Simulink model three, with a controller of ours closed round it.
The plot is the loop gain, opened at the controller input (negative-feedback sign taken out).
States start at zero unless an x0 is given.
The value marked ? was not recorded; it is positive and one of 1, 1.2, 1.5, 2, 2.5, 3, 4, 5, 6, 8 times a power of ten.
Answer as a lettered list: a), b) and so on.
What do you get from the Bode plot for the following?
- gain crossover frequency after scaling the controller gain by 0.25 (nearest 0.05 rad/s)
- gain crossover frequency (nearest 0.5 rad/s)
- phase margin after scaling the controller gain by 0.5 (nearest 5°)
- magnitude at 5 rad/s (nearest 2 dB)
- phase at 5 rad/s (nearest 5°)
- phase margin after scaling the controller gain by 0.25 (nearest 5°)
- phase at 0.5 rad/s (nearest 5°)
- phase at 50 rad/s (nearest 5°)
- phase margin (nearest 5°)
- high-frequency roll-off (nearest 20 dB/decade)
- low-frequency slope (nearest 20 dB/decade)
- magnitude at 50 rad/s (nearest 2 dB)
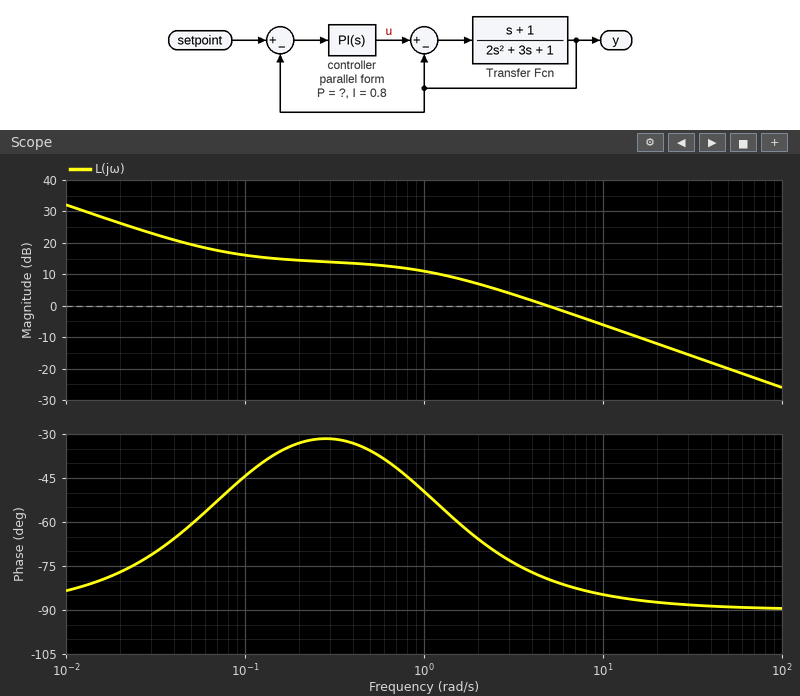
a) 0.75 rad/s
b) 5.0 rad/s
c) 110°
d) 0 dB
e) -80°
f) 135°
g) -35°
h) -90°
i) 100°
j) -20 dB/decade
k) -20 dB/decade
l) -20 dB
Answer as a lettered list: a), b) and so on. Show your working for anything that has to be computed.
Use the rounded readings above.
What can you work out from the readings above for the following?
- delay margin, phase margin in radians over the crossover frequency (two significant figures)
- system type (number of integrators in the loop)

a) 100 × π / 180 / 5 = 0.35 s
b) 1
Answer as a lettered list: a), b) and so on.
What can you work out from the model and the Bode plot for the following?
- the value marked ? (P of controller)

a) 10
